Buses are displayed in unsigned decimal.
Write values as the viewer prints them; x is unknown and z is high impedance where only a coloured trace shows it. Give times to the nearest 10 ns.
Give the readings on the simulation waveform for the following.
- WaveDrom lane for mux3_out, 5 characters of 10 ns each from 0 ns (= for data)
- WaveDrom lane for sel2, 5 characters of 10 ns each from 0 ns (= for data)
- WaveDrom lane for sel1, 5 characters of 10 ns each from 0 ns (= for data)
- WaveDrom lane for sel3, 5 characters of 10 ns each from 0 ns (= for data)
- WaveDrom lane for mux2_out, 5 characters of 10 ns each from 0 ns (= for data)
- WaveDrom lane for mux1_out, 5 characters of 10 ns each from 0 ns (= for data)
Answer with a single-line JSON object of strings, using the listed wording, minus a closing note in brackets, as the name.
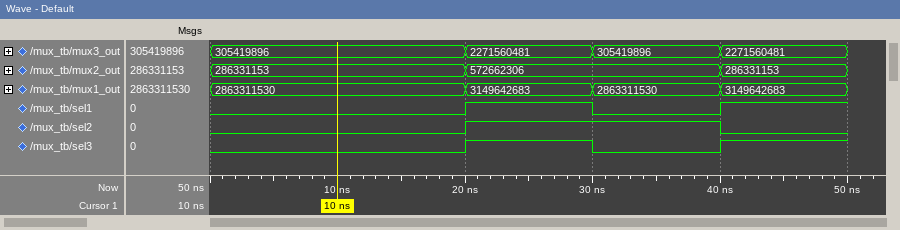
{"WaveDrom lane for mux3_out, 5 characters of 10 ns each from 0 ns": "{name: 'mux3_out', wave: '=.===', data: '305419896 2271560481 305419896 2271560481'}", "WaveDrom lane for sel2, 5 characters of 10 ns each from 0 ns": "{name: 'sel2', wave: '0.1.0'}", "WaveDrom lane for sel1, 5 characters of 10 ns each from 0 ns": "{name: 'sel1', wave: '0.101'}", "WaveDrom lane for sel3, 5 characters of 10 ns each from 0 ns": "{name: 'sel3', wave: '0.101'}", "WaveDrom lane for mux2_out, 5 characters of 10 ns each from 0 ns": "{name: 'mux2_out', wave: '=.=.=', data: '286331153 572662306 286331153'}", "WaveDrom lane for mux1_out, 5 characters of 10 ns each from 0 ns": "{name: 'mux1_out', wave: '=.===', data: '2863311530 3149642683 2863311530 3149642683'}"}
